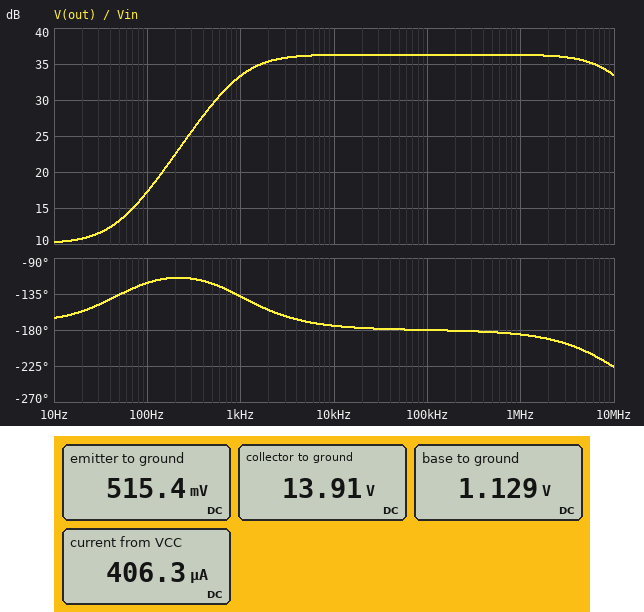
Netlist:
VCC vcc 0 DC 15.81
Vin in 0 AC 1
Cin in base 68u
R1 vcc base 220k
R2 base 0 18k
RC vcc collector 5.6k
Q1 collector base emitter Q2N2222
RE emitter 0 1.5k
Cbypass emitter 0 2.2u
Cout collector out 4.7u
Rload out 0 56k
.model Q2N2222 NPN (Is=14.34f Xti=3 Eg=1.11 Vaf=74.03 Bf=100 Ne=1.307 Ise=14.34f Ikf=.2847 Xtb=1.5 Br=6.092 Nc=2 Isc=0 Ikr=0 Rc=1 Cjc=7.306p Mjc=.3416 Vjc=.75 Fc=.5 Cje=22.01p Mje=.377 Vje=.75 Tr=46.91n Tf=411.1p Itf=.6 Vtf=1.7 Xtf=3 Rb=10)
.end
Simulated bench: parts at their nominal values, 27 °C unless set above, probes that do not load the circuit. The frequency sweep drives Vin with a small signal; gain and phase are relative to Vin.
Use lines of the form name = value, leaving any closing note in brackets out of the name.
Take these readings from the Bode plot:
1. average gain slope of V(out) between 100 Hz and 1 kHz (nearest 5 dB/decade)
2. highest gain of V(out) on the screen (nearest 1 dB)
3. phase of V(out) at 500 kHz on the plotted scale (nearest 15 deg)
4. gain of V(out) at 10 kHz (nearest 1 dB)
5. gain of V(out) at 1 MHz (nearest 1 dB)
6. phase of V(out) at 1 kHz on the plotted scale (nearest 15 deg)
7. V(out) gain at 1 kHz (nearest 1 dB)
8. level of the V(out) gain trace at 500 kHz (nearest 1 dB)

average gain slope of V(out) between 100 Hz and 1 kHz = 15 dB/decade
highest gain of V(out) on the screen = 36 dB
phase of V(out) at 500 kHz on the plotted scale = -180 deg
gain of V(out) at 10 kHz = 36 dB
gain of V(out) at 1 MHz = 36 dB
phase of V(out) at 1 kHz on the plotted scale = -135 deg
V(out) gain at 1 kHz = 33 dB
level of the V(out) gain trace at 500 kHz = 36 dB
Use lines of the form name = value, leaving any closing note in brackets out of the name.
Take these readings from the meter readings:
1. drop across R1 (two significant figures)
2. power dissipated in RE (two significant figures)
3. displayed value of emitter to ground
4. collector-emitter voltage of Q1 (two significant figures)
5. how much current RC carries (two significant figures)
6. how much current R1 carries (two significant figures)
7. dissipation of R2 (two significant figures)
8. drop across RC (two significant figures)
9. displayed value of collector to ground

drop across R1 = 15 V
power dissipated in RE = 180 µW
displayed value of emitter to ground = 515.4 mV
collector-emitter voltage of Q1 = 13 V
how much current RC carries = 340 µA
how much current R1 carries = 67 µA
dissipation of R2 = 71 µW
drop across RC = 1.9 V
displayed value of collector to ground = 13.91 V
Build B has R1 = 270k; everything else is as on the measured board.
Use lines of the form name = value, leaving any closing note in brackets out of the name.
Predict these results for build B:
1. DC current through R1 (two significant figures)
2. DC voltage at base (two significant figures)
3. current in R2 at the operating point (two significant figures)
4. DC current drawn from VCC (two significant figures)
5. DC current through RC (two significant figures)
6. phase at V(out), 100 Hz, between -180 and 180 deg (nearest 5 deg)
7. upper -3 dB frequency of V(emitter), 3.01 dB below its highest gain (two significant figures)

DC current through R1 = 55 µA
DC voltage at base = 940 mV
current in R2 at the operating point = 52 µA
DC current drawn from VCC = 280 µA
DC current through RC = 220 µA
phase at V(out), 100 Hz, between -180 and 180 deg = -125 deg
upper -3 dB frequency of V(emitter), 3.01 dB below its highest gain = 670 Hz
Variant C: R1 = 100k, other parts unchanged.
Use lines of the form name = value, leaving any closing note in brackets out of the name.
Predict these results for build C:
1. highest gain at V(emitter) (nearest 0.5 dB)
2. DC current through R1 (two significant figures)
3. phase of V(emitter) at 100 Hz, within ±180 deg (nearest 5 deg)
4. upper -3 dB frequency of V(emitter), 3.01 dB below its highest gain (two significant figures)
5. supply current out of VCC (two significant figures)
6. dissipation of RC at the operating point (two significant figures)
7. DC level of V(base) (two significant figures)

highest gain at V(emitter) = 0 dB
DC current through R1 = 140 µA
phase of V(emitter) at 100 Hz, within ±180 deg = 0 deg
upper -3 dB frequency of V(emitter), 3.01 dB below its highest gain = 2.8 kHz
supply current out of VCC = 1.2 mA
dissipation of RC at the operating point = 6.1 mW
DC level of V(base) = 2.2 V
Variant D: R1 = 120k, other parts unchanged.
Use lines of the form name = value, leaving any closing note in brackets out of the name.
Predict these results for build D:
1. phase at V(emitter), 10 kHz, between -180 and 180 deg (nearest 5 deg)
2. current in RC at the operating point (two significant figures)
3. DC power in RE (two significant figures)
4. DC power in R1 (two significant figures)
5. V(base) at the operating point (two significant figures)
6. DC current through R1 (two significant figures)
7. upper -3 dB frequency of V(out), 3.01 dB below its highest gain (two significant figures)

phase at V(emitter), 10 kHz, between -180 and 180 deg = -75 deg
current in RC at the operating point = 840 µA
DC power in RE = 1.1 mW
DC power in R1 = 1.6 mW
V(base) at the operating point = 1.9 V
DC current through R1 = 120 µA
upper -3 dB frequency of V(out), 3.01 dB below its highest gain = 8.2 MHz
